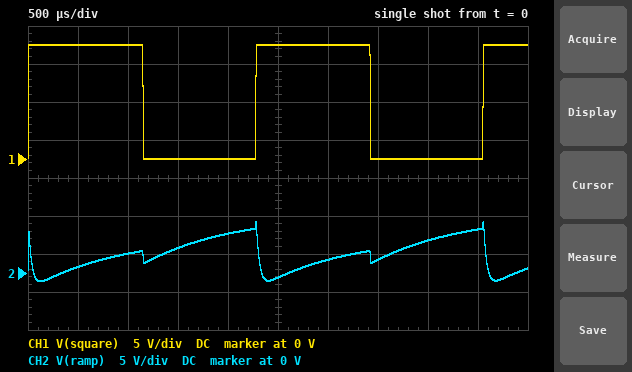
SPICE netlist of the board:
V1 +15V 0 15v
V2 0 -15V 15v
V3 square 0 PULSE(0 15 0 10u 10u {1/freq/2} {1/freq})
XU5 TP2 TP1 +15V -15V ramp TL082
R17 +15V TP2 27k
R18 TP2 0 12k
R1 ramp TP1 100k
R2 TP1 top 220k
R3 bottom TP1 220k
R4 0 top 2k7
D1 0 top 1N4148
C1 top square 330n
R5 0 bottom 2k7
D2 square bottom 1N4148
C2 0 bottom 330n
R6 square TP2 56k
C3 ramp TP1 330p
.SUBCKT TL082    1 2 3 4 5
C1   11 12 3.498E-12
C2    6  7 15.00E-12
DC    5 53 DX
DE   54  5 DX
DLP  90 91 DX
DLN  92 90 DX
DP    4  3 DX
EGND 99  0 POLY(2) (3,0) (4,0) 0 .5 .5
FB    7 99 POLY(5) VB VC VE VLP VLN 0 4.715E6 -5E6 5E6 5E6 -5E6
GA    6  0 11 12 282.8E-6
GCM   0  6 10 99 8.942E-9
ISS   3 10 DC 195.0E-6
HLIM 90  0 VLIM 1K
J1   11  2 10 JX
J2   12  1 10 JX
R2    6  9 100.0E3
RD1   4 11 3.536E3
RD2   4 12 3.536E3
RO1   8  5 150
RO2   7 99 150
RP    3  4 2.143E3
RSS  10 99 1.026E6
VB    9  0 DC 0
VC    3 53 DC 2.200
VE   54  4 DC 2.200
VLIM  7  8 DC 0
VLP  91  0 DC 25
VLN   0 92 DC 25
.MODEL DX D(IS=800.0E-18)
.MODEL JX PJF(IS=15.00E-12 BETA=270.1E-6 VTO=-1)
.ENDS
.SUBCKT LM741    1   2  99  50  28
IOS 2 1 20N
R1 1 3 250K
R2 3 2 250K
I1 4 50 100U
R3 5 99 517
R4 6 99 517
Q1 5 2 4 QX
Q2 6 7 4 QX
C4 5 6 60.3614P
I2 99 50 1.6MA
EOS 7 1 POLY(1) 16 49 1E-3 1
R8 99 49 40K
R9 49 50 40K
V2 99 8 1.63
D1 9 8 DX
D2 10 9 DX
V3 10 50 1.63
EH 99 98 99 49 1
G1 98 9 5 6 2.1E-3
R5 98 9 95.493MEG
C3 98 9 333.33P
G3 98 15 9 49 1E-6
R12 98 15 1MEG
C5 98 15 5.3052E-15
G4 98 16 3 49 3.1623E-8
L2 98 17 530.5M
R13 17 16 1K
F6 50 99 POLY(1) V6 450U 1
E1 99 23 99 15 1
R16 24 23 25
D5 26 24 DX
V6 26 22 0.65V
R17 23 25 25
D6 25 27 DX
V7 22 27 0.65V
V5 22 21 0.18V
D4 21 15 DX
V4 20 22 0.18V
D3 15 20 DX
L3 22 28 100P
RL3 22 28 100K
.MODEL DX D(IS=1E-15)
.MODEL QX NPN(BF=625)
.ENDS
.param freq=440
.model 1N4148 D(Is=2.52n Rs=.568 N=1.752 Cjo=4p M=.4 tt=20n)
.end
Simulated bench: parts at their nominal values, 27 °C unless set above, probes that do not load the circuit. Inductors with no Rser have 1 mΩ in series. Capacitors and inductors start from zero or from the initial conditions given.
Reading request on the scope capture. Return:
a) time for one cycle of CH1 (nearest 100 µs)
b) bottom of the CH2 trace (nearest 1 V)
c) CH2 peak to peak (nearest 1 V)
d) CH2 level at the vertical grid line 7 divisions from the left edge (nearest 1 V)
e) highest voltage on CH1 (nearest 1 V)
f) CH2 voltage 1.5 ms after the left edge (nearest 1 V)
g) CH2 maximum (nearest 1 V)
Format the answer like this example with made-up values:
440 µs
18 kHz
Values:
2.3 ms
-1 V
8 V
2 V
15 V
3 V
7 V
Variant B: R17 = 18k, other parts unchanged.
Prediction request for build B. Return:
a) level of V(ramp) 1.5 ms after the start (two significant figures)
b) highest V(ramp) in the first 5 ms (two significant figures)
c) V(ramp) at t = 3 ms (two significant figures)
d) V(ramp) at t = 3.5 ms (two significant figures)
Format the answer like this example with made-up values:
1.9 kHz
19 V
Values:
5.8 V
9.0 V
3.8 V
4.2 V
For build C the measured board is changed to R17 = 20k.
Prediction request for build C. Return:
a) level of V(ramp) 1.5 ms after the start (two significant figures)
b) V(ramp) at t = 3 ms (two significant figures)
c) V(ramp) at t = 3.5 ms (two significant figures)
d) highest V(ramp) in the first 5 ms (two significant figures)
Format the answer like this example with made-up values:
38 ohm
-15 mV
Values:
5.1 V
3.2 V
3.5 V
8.4 V
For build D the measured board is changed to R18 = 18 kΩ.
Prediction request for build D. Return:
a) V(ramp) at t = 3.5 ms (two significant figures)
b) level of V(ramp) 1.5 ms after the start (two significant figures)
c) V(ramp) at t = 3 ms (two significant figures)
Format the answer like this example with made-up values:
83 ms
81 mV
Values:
3.7 V
5.2 V
4.6 V
